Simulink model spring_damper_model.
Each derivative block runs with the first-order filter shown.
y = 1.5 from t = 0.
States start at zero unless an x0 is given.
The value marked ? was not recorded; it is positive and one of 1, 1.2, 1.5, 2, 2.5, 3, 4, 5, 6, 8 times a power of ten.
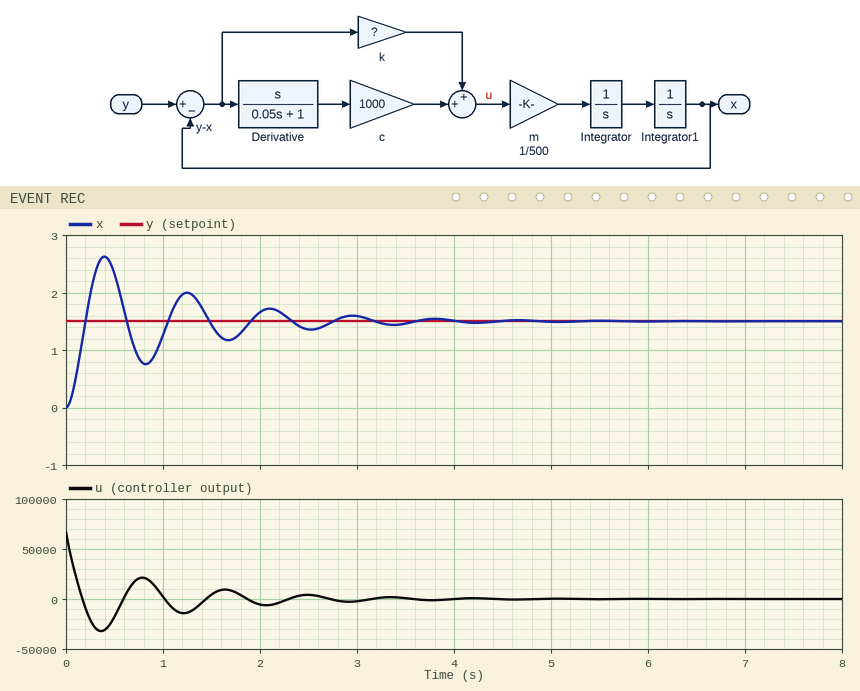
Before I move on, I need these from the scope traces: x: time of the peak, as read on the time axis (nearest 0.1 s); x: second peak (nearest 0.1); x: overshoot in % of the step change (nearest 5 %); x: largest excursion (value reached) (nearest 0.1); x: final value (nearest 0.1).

0.4 s
2.0
75 %
2.6
1.5
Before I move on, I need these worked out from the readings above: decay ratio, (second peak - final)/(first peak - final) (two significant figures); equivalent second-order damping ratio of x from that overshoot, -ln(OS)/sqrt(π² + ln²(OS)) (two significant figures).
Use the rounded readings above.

0.45
0.091
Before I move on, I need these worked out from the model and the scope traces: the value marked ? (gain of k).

25000
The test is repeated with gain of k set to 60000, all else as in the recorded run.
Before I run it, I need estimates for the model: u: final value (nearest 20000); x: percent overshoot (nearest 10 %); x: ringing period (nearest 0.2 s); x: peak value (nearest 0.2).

0
90 %
0.6 s
2.8
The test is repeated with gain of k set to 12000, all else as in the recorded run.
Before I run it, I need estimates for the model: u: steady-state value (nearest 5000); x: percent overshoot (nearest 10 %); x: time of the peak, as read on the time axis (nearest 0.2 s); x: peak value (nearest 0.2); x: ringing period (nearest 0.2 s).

0
60 %
0.6 s
2.4
1.2 s
